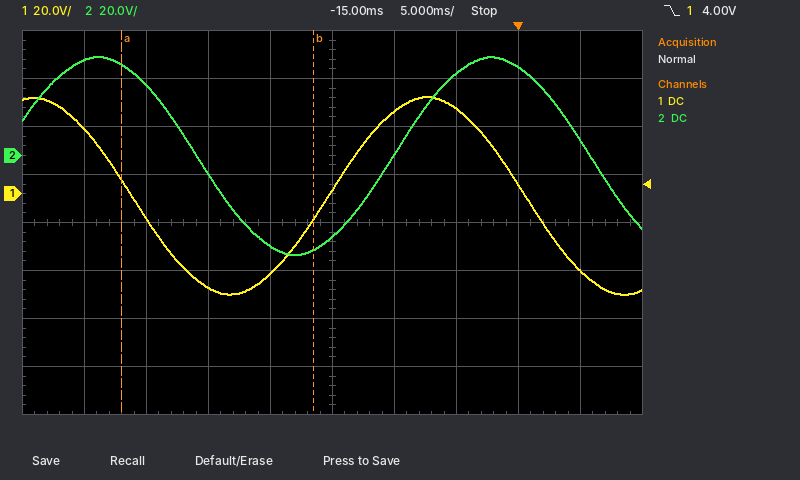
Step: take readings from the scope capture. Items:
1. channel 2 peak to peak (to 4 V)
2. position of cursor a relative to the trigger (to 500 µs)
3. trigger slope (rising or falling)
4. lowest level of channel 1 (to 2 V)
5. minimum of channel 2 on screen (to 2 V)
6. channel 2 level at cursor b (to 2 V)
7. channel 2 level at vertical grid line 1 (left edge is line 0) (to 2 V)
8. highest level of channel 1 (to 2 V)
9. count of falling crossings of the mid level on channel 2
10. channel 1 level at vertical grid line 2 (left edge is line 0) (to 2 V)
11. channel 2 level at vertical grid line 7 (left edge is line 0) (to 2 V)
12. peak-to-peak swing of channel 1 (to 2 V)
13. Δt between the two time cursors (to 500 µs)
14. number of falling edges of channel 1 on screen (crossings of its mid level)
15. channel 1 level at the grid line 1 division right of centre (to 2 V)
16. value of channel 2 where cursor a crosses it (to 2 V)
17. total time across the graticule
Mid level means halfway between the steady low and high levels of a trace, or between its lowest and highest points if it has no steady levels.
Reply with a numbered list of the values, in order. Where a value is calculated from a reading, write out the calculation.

1. 84 V
2. -32.0 ms
3. falling
4. -42 V
5. -42 V
6. -40 V
7. 40 V
8. 40 V
9. 2
10. -10 V
11. 34 V
12. 40 V − (-42 V) = 82 V
13. 15.5 ms
14. 2
15. 34 V
16. 38 V
17. 50 ms
